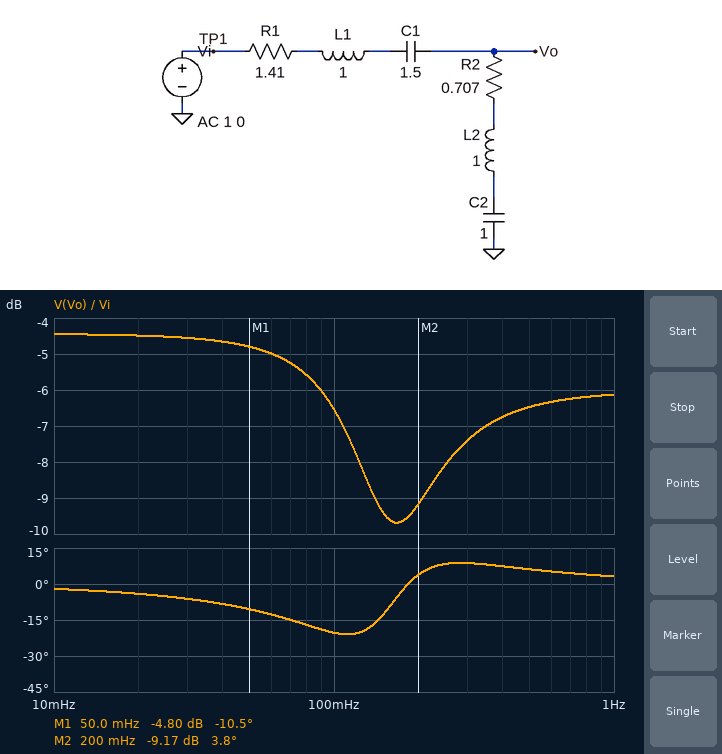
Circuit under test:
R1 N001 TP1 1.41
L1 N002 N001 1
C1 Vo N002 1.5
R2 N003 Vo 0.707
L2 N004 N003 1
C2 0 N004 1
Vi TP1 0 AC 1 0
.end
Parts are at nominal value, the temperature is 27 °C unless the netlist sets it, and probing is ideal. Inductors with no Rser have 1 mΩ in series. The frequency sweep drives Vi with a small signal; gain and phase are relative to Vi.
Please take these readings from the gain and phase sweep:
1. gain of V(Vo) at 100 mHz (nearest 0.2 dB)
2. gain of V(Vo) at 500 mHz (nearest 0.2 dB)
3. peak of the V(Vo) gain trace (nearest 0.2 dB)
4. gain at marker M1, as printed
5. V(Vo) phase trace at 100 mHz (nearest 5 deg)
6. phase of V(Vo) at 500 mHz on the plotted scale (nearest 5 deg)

-6.6 dB
-6.4 dB
-4.4 dB
-4.80 dB
-20 deg
5 deg
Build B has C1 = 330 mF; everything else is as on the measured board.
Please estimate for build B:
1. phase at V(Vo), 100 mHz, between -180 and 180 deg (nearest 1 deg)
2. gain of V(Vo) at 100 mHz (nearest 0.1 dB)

14 deg
-13.4 dB
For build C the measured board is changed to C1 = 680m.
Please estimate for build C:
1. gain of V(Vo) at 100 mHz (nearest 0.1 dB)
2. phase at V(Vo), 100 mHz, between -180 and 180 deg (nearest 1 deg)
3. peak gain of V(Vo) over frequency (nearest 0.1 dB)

-9.1 dB
-2 deg
-6.0 dB
